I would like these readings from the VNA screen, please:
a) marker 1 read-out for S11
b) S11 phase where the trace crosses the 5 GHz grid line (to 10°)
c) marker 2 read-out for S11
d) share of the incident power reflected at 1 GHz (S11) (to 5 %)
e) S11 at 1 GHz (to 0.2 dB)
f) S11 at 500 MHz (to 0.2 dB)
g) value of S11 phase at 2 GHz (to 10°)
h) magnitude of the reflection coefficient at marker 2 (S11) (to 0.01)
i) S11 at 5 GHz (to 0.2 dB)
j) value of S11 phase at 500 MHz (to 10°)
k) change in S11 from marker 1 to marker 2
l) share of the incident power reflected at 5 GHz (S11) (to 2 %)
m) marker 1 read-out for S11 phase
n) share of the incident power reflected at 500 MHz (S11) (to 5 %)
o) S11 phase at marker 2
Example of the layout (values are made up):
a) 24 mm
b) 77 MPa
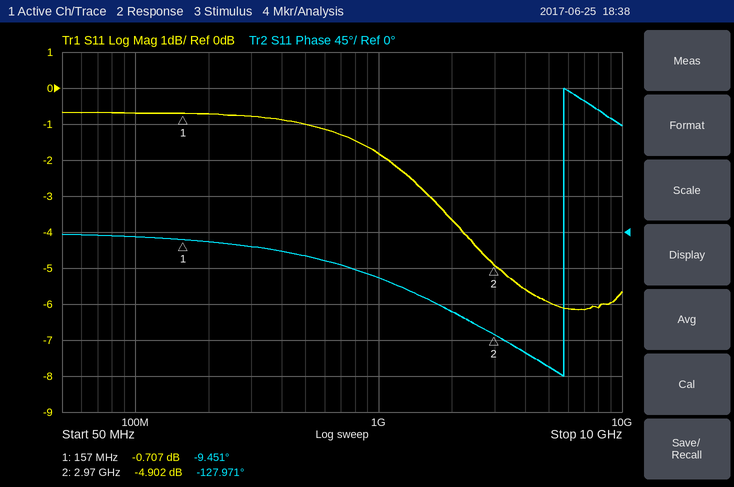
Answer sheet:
a) -0.707 dB
b) -170°
c) -4.902 dB
d) 65 %
e) -1.8 dB
f) -1.0 dB
g) -100°
h) 0.57
i) -6.0 dB
j) -30°
k) -4.195 dB
l) 26 %
m) -9.451°
n) 80 %
o) -127.971°
